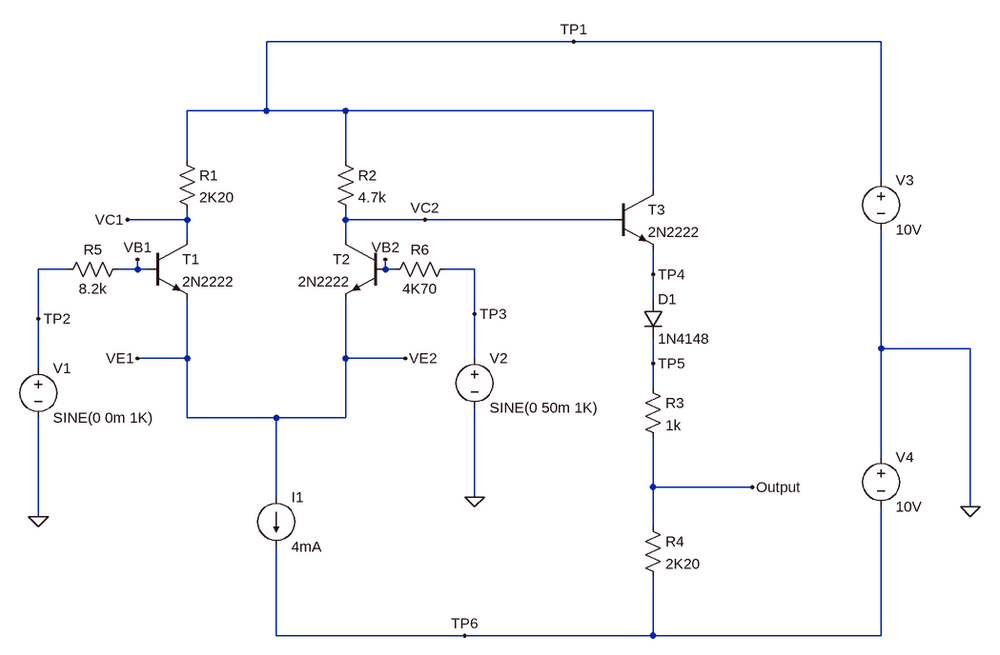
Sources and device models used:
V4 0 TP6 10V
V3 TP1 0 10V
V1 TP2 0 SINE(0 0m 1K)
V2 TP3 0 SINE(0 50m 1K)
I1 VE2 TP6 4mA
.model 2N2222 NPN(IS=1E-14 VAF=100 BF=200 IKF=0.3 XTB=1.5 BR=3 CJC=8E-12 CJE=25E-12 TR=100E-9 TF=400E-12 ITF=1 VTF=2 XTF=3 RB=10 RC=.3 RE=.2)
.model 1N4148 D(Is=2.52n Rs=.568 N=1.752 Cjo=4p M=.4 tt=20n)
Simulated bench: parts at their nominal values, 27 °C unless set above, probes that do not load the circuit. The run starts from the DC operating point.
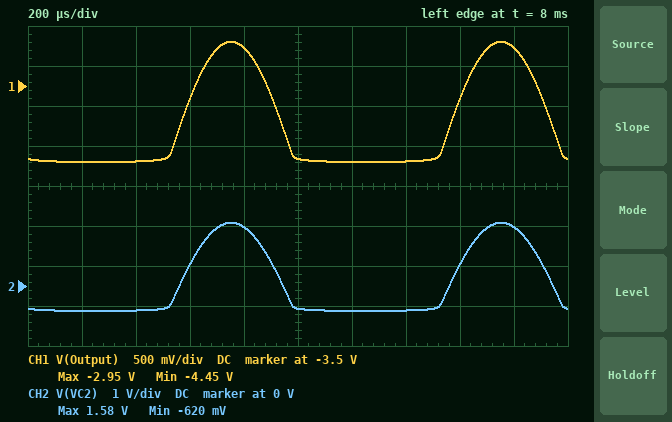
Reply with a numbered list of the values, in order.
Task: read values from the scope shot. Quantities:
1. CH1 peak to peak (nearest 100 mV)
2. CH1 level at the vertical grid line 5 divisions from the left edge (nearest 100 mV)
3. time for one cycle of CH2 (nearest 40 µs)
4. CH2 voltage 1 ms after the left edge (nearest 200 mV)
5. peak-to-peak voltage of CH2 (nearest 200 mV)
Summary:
1. 1.5 V
2. -4.4 V
3. 1.00 ms
4. -600 mV
5. 2.2 V
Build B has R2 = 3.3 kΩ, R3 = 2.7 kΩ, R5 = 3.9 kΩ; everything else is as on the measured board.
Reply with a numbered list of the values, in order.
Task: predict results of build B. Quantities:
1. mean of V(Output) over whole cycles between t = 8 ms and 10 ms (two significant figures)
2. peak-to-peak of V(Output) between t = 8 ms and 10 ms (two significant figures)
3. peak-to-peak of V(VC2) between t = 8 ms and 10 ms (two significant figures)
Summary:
1. -4.4 V
2. 2.0 V
3. 4.5 V
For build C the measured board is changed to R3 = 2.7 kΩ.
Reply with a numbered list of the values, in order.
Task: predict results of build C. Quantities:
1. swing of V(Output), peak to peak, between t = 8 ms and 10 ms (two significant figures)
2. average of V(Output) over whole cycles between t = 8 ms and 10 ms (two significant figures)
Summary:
1. 990 mV
2. -6.1 V
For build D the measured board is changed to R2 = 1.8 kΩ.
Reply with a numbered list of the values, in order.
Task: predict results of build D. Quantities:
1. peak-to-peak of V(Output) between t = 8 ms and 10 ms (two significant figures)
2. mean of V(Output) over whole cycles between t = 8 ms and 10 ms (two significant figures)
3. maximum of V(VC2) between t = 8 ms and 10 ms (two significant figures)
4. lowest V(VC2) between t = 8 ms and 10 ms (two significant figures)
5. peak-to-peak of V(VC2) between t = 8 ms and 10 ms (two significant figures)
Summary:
1. 1.3 V
2. -120 mV
3. 6.7 V
4. 4.8 V
5. 1.9 V
